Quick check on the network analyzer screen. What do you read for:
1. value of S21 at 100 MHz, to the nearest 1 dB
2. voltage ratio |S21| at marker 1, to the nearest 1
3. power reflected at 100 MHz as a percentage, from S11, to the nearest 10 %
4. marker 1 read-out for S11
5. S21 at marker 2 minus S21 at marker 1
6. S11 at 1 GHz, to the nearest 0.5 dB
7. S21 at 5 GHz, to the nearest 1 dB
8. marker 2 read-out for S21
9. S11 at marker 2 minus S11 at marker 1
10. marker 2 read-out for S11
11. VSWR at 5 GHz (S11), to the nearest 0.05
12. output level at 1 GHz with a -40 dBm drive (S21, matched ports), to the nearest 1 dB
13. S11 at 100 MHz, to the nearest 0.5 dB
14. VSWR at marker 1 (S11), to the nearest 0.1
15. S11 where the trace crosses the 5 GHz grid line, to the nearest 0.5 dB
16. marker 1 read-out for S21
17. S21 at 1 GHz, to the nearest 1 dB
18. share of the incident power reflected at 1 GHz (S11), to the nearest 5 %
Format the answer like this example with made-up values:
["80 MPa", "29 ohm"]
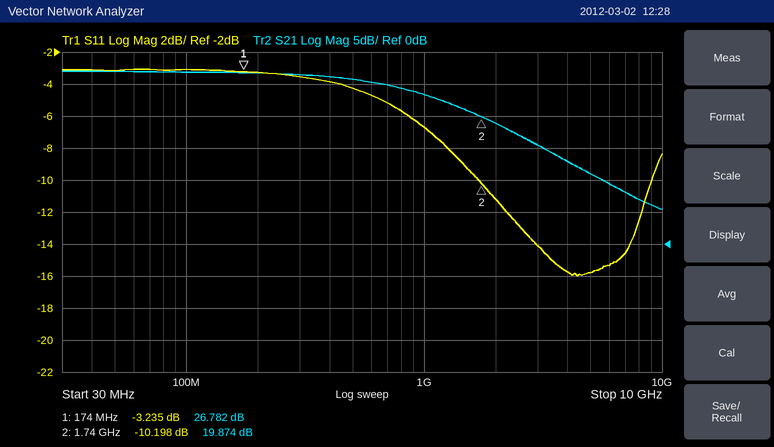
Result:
["27 dB", "22", "50 %", "-3.235 dB", "-6.908 dB", "-6.5 dB", "11 dB", "19.874 dB", "-6.963 dB", "-10.198 dB", "1.40", "-17 dBm", "-3.0 dB", "5.4", "-16.0 dB", "26.782 dB", "23 dB", "20 %"]
